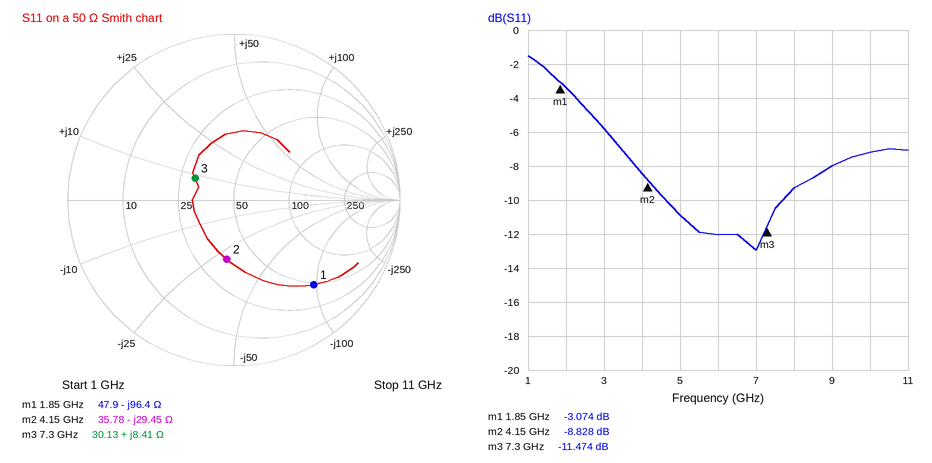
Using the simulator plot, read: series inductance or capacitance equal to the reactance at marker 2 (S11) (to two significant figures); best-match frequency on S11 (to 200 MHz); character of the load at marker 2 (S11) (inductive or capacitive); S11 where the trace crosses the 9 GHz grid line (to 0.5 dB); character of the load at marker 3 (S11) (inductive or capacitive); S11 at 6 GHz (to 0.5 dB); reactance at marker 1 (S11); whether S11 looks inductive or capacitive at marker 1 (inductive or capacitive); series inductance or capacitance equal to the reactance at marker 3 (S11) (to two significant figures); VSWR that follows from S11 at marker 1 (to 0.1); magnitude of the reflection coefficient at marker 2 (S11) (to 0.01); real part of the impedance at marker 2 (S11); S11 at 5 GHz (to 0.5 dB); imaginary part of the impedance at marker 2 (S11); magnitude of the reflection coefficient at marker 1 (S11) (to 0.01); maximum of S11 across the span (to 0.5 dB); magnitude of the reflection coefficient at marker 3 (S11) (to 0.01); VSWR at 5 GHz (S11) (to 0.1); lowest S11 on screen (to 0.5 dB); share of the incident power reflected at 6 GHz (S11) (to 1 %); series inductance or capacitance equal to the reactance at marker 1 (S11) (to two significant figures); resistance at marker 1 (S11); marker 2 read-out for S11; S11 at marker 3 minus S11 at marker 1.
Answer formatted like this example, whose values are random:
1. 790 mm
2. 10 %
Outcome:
1. 1.3 pF
2. 7.0 GHz
3. capacitive
4. -8.0 dB
5. inductive
6. -12.0 dB
7. -96.4 Ω
8. capacitive
9. 180 pH
10. 5.7
11. 0.36
12. 35.78 Ω
13. -11.0 dB
14. -29.45 Ω
15. 0.70
16. -1.5 dB
17. 0.27
18. 1.8
19. -13.0 dB
20. 6 %
21. 890 fF
22. 47.9 Ω
23. -8.828 dB
24. -8.400 dB
